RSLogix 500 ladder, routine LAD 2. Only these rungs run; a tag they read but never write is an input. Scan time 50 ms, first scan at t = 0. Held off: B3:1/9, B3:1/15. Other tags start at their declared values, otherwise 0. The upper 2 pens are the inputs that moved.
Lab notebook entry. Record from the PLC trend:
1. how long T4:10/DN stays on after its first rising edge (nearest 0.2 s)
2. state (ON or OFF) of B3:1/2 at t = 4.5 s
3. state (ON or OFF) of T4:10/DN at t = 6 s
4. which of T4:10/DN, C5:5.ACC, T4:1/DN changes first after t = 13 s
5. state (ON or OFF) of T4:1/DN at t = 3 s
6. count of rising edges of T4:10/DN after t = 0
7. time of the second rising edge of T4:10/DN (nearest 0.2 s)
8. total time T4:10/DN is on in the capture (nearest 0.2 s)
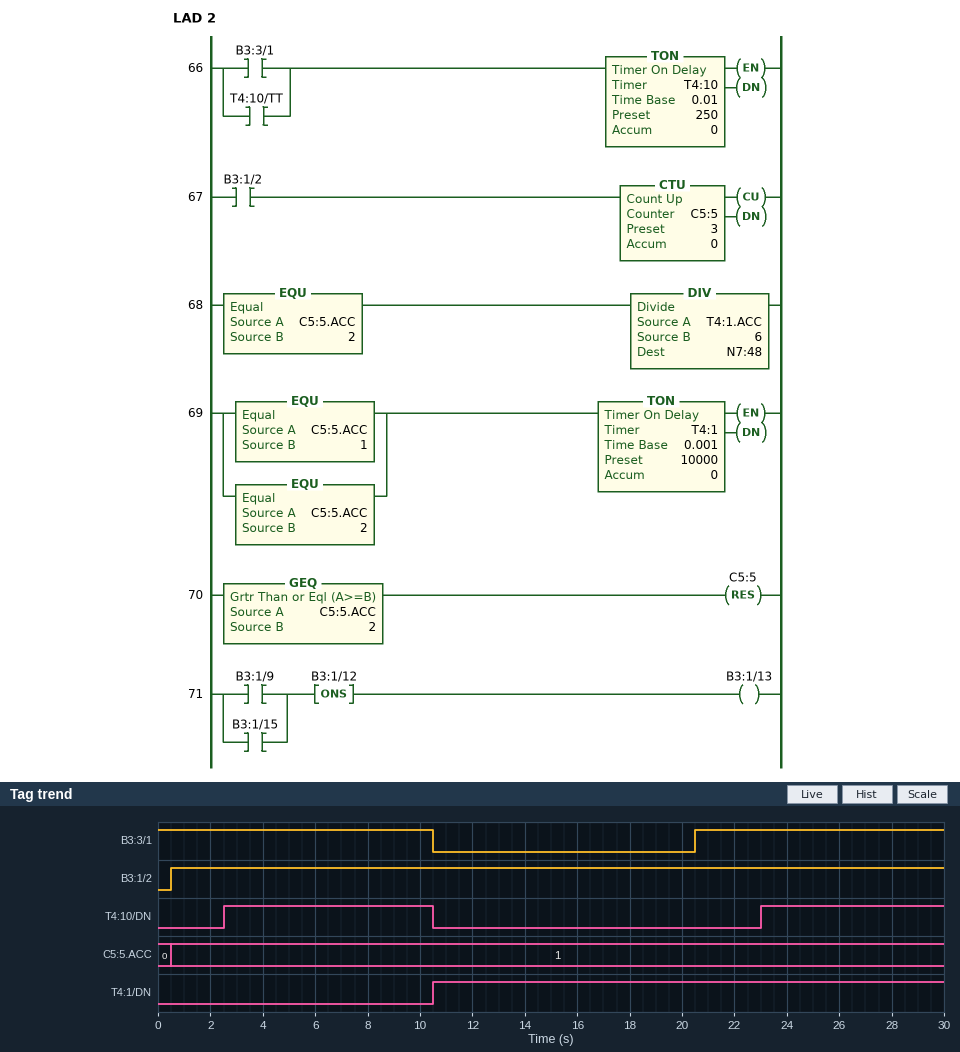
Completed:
8.0 s
ON
ON
T4:10/DN
OFF
2
23.0 s
15.0 s
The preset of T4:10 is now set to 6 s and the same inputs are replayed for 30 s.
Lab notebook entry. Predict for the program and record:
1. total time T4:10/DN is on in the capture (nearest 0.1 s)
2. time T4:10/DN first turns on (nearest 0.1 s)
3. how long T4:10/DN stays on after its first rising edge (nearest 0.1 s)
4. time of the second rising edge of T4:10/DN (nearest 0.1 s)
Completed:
8.0 s
6.0 s
4.5 s
26.5 s
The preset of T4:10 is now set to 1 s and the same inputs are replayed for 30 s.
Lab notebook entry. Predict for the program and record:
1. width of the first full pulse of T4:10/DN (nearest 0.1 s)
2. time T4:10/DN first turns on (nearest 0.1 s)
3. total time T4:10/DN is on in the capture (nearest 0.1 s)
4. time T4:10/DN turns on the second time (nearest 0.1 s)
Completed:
9.5 s
1.0 s
18.0 s
21.5 s
